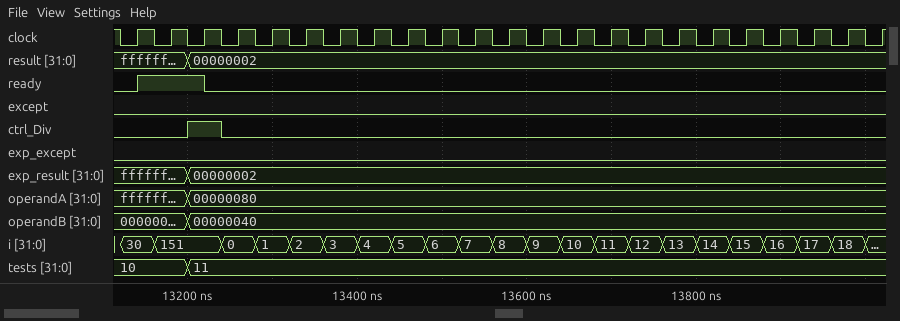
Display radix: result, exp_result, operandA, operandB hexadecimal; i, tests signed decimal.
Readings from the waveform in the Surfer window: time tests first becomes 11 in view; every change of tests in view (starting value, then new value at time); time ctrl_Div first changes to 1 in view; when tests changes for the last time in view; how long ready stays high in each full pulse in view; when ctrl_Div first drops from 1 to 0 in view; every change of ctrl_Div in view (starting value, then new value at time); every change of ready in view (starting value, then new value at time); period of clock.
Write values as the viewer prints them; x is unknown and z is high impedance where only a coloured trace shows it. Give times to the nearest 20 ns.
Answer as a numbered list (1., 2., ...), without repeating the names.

1. 13200 ns
2. 10, 11 at 13200 ns
3. 13200 ns
4. 13200 ns
5. 80 ns
6. 13240 ns
7. 0, 1 at 13200 ns, 0 at 13240 ns
8. 0, 1 at 13140 ns, 0 at 13220 ns
9. 40 ns
